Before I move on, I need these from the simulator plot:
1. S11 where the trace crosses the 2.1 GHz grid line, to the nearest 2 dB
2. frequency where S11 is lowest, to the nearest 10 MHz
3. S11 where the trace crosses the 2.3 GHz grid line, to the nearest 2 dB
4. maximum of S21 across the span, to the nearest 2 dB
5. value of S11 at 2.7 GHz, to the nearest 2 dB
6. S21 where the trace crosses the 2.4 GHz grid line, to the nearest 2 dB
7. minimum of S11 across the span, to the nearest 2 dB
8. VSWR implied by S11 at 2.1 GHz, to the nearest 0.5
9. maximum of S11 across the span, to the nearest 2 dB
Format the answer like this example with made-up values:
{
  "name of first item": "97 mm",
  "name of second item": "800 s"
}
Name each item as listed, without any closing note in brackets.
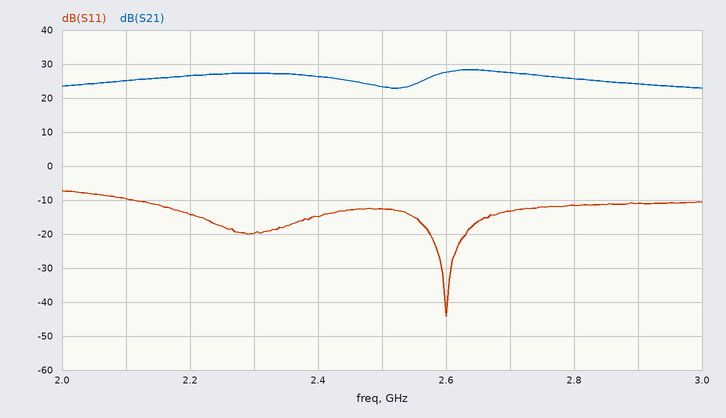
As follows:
{
  "S11 where the trace crosses the 2.1 GHz grid line, to the nearest 2 dB": "-10 dB",
  "frequency where S11 is lowest, to the nearest 10 MHz": "2.60 GHz",
  "S11 where the trace crosses the 2.3 GHz grid line, to the nearest 2 dB": "-20 dB",
  "maximum of S21 across the span, to the nearest 2 dB": "28 dB",
  "value of S11 at 2.7 GHz, to the nearest 2 dB": "-14 dB",
  "S21 where the trace crosses the 2.4 GHz grid line, to the nearest 2 dB": "26 dB",
  "minimum of S11 across the span, to the nearest 2 dB": "-44 dB",
  "VSWR implied by S11 at 2.1 GHz, to the nearest 0.5": "2.0",
  "maximum of S11 across the span, to the nearest 2 dB": "-8 dB"
}
